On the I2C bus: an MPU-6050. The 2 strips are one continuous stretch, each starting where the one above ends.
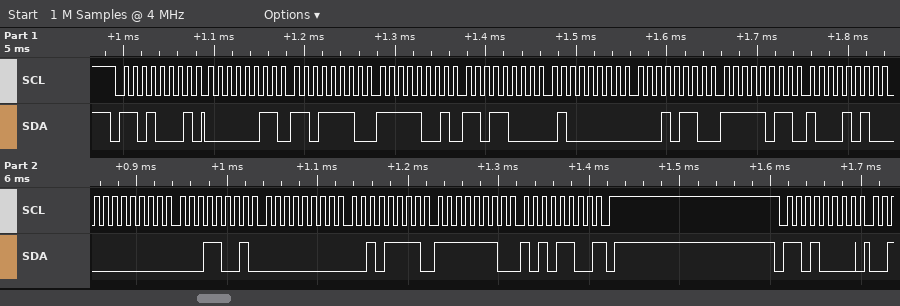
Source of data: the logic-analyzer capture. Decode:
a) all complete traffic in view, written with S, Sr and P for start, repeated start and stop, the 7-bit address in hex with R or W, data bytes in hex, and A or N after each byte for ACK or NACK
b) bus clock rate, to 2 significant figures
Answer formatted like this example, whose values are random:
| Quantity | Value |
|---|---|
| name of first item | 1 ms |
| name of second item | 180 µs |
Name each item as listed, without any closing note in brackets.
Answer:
| Quantity | Value |
|---|---|
| all complete traffic in view, written with S, Sr and P for start, repeated start and stop, the 7-bit address in hex with R or W, data bytes in hex, and A or N after each byte for ACK or NACK | S 68R A 03 A DE A F9 A D8 A 40 A 16 A FB A 8A A 00 A 19 A 00 A 2F A FE A AC N P S 68W A |
| bus clock rate, to 2 significant figures | 100 kHz |
